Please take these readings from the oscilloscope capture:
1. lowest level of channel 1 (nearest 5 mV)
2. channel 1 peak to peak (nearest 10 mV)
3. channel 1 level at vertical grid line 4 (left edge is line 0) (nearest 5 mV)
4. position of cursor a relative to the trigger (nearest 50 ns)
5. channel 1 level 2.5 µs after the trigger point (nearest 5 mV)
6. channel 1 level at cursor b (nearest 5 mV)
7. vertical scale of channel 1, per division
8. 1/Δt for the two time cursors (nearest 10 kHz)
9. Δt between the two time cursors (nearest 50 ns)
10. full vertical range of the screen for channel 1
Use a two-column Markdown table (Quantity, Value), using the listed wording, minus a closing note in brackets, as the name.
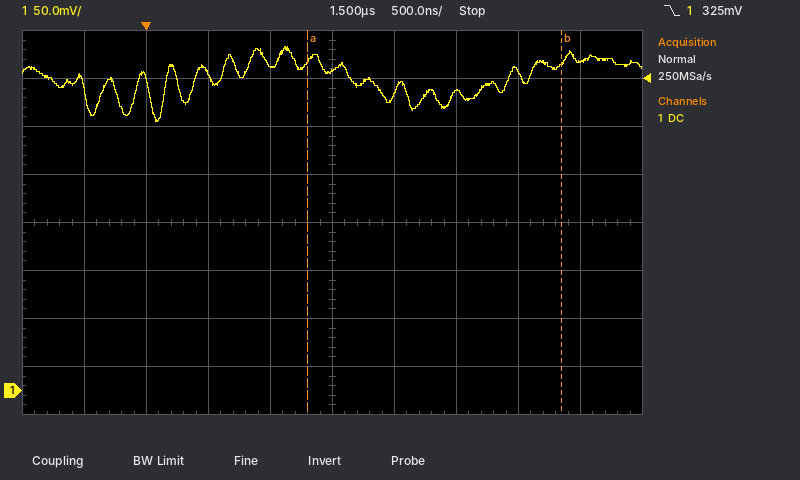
| Quantity | Value |
|---|---|
| lowest level of channel 1 | 280 mV |
| channel 1 peak to peak | 80 mV |
| channel 1 level at vertical grid line 4 (left edge is line 0) | 340 mV |
| position of cursor a relative to the trigger | +1.30 µs |
| channel 1 level 2.5 µs after the trigger point | 310 mV |
| channel 1 level at cursor b | 340 mV |
| vertical scale of channel 1, per division | 50 mV |
| 1/Δt for the two time cursors | 490 kHz |
| Δt between the two time cursors | 2.05 µs |
| full vertical range of the screen for channel 1 | 400 mV |
